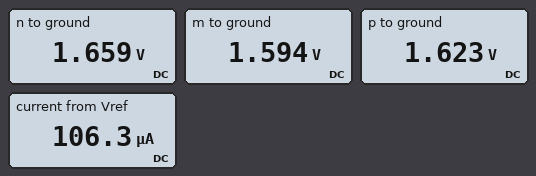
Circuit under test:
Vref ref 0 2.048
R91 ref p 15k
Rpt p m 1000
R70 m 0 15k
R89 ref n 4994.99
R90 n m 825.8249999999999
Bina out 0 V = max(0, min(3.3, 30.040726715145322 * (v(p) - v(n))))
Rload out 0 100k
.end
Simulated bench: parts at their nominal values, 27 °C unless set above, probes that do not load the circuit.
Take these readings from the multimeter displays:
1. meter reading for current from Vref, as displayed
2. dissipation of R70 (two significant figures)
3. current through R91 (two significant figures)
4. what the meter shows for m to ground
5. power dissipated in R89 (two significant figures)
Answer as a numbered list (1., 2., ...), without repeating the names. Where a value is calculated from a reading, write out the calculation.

1. 106.3 µA
2. (1.594 V)^2 / 15 kΩ = 170 µW
3. (2.048 V - 1.623 V) / 15 kΩ = 28 µA
4. 1.594 V
5. (2.048 V - 1.659 V)^2 / 4.995 kΩ = 30 µW
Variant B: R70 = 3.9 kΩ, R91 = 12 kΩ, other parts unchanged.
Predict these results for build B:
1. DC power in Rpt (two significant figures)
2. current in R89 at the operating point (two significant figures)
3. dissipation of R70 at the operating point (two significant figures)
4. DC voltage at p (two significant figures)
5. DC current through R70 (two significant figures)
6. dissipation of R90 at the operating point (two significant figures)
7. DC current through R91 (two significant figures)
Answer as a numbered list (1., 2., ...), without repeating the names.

1. 6.4 µW
2. 180 µA
3. 260 µW
4. 1.1 V
5. 260 µA
6. 26 µW
7. 80 µA
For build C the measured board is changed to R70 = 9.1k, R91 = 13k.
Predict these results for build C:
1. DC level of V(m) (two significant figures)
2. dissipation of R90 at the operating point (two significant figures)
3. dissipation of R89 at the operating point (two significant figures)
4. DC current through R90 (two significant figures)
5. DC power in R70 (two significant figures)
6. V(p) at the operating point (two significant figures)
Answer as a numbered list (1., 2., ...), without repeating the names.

1. 1.4 V
2. 9.9 µW
3. 60 µW
4. 110 µA
5. 220 µW
6. 1.5 V
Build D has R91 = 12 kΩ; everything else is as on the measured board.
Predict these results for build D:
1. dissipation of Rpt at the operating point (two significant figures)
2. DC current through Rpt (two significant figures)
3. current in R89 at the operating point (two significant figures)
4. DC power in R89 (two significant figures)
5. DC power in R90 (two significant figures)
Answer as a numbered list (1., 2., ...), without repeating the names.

1. 1.1 µW
2. 33 µA
3. 74 µA
4. 28 µW
5. 4.6 µW
